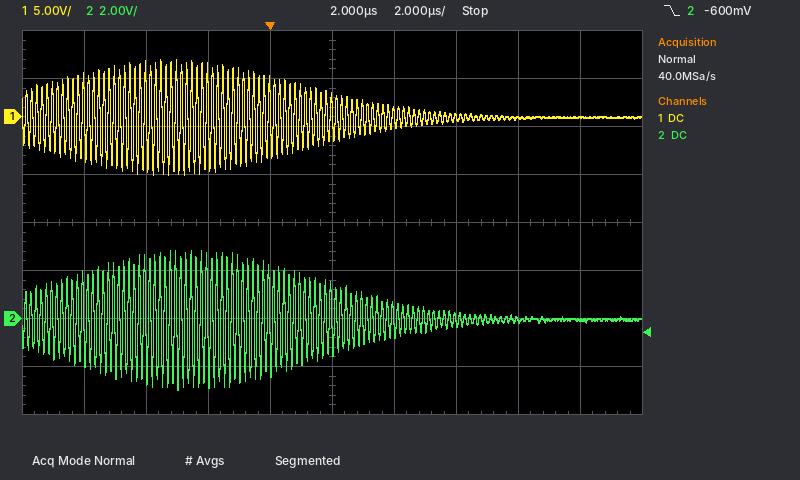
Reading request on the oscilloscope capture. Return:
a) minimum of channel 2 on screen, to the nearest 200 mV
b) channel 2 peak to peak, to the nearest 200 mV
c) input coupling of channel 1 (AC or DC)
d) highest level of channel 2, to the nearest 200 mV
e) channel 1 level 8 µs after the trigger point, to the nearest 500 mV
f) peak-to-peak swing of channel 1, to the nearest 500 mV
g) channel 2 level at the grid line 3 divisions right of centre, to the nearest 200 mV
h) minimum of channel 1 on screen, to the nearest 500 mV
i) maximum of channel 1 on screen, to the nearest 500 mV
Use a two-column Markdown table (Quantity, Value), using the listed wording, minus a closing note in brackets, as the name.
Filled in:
| Quantity | Value |
|---|---|
| minimum of channel 2 on screen, to the nearest 200 mV | -3.0 V |
| channel 2 peak to peak, to the nearest 200 mV | 5.8 V |
| input coupling of channel 1 | DC |
| highest level of channel 2, to the nearest 200 mV | 2.8 V |
| channel 1 level 8 µs after the trigger point, to the nearest 500 mV | 0.0 V |
| peak-to-peak swing of channel 1, to the nearest 500 mV | 12.0 V |
| channel 2 level at the grid line 3 divisions right of centre, to the nearest 200 mV | 0.0 V |
| minimum of channel 1 on screen, to the nearest 500 mV | -6.0 V |
| maximum of channel 1 on screen, to the nearest 500 mV | 6.0 V |
